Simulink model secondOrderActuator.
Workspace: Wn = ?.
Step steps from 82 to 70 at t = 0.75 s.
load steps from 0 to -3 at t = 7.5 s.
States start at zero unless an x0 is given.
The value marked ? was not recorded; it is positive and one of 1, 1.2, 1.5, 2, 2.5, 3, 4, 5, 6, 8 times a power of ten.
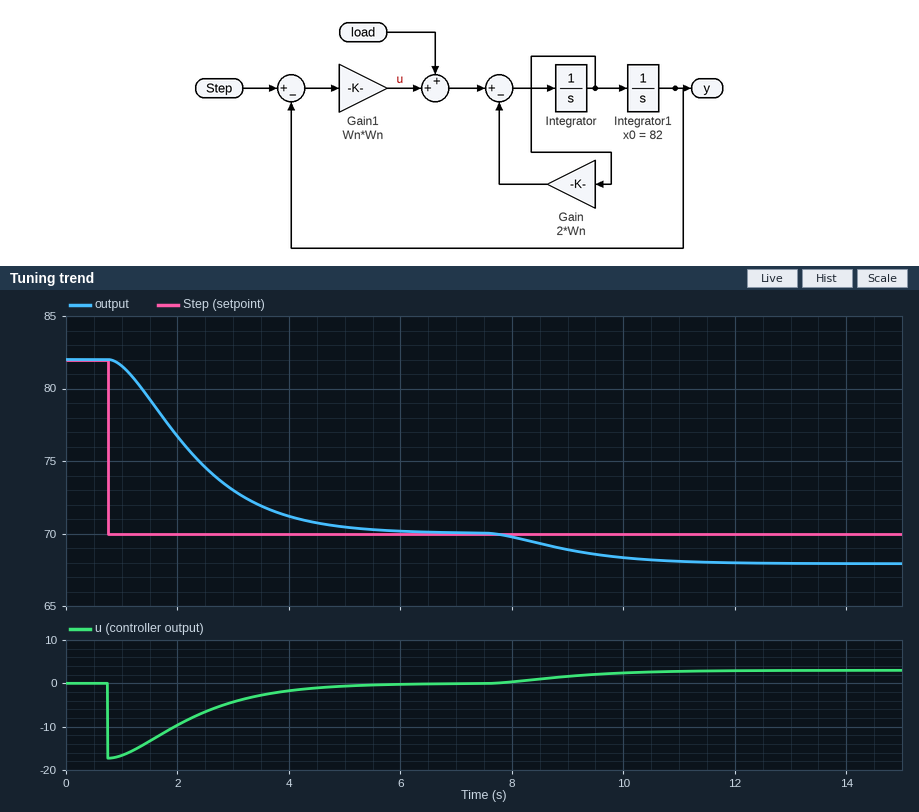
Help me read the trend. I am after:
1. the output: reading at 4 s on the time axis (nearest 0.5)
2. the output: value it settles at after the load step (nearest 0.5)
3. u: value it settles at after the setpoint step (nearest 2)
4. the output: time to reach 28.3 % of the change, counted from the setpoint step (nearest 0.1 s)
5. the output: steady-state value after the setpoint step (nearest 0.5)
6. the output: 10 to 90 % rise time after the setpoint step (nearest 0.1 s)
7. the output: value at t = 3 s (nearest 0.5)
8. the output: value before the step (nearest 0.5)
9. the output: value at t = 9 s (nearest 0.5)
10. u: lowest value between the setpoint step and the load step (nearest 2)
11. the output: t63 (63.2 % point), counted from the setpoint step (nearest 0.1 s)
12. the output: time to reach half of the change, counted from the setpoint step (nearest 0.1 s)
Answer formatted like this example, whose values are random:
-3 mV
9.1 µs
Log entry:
71.0
68.0
0
0.9 s
70.0
2.8 s
73.0
82.0
69.0
-18
1.8 s
1.4 s
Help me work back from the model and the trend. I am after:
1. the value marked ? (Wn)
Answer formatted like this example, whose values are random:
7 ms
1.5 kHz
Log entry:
1.2
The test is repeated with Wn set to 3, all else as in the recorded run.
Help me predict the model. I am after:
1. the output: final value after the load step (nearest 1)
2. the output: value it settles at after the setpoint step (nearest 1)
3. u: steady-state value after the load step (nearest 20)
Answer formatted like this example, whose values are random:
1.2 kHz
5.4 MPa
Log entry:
70
70
0
